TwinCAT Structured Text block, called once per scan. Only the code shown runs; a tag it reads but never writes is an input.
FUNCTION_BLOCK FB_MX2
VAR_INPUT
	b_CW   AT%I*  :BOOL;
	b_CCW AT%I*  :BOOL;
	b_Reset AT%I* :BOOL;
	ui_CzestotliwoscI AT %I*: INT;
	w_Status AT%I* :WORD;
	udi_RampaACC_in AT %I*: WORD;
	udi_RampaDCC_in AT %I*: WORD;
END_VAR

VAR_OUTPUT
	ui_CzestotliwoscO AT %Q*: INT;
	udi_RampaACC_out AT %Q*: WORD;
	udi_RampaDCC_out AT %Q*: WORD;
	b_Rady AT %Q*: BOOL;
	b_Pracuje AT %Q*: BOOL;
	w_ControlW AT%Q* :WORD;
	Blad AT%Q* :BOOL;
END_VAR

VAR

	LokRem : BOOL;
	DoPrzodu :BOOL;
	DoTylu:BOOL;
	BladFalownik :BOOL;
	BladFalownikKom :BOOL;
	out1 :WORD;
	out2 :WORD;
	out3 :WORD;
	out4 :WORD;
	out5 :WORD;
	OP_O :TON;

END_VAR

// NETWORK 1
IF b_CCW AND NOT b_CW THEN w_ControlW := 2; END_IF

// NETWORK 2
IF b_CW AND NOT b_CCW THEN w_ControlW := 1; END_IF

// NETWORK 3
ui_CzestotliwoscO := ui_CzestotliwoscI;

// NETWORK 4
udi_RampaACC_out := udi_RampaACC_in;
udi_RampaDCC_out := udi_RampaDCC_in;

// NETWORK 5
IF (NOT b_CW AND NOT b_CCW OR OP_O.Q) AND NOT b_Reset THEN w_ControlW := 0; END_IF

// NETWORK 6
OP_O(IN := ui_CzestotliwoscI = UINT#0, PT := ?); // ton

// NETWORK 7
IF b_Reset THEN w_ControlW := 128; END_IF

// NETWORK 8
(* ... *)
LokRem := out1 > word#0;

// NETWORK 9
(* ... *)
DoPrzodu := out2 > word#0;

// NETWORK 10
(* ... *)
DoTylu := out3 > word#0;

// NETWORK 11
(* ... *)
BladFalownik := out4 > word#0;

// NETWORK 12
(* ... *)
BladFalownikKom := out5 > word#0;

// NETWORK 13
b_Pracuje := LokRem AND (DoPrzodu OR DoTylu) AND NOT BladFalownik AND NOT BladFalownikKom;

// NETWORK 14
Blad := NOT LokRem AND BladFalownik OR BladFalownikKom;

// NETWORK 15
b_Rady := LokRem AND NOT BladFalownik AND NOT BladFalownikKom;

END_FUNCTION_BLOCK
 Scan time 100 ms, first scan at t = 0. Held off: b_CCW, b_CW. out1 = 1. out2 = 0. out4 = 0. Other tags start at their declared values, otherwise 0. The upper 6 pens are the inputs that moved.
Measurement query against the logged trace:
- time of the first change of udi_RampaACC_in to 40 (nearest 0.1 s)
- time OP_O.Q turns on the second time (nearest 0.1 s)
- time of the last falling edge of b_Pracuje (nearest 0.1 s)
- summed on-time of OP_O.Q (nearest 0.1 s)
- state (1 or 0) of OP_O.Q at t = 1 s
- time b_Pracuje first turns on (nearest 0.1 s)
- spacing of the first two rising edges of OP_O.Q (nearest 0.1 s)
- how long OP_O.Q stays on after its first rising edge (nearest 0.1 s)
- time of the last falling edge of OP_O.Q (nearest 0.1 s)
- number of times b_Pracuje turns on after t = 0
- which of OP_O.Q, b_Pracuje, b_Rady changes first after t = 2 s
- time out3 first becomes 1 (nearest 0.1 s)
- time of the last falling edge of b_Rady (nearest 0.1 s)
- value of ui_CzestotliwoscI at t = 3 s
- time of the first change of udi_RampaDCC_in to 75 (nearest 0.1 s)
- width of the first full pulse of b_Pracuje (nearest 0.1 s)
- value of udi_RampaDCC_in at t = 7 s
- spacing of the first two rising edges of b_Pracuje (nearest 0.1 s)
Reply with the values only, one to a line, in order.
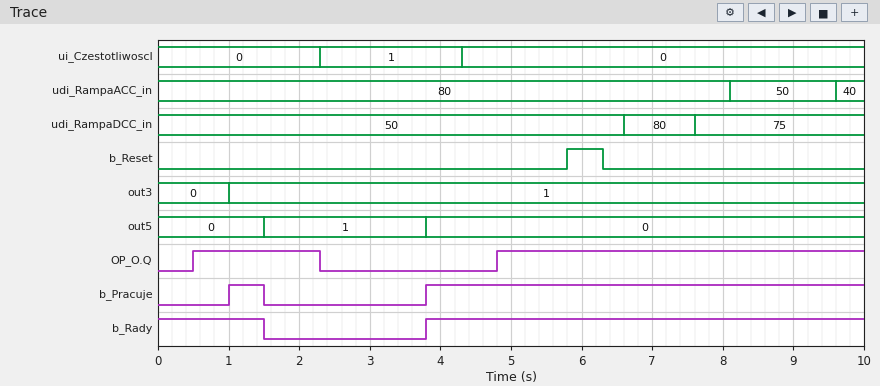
9.6 s
4.8 s
1.5 s
7.0 s
1
1.0 s
4.3 s
1.8 s
2.3 s
2
OP_O.Q
1.0 s
1.5 s
1
7.6 s
0.5 s
80
2.8 s
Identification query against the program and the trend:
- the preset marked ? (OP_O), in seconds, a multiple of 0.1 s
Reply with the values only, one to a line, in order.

0.5 s
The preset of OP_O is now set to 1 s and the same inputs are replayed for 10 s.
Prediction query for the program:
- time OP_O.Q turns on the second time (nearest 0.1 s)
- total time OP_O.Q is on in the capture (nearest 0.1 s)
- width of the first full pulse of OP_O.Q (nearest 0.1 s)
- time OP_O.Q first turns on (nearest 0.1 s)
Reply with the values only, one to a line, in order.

5.3 s
6.0 s
1.3 s
1.0 s
